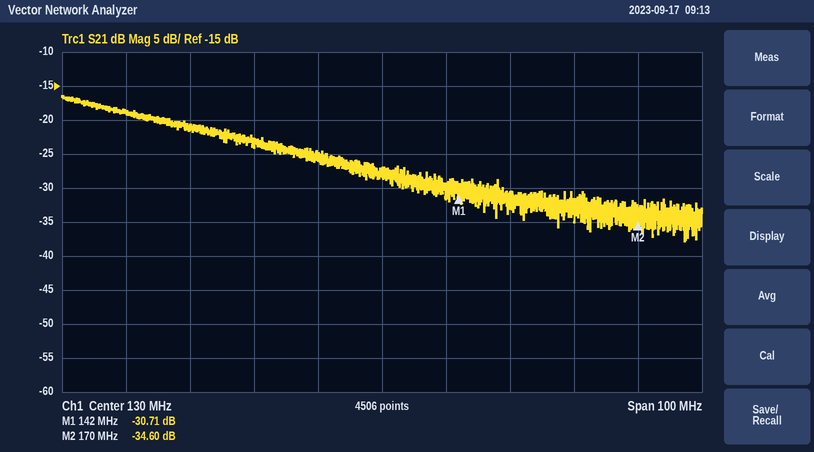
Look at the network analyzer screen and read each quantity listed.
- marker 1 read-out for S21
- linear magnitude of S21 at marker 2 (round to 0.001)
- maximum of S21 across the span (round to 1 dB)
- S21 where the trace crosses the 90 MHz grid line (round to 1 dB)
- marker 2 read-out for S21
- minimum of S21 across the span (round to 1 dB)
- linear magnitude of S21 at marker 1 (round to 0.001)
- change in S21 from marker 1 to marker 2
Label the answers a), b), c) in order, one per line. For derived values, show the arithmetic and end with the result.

a) -30.71 dB
b) 10^(-34.6/20) ≈ 0.019
c) -16 dB
d) -19 dB
e) -34.60 dB
f) -38 dB
g) 10^(-30.71/20) ≈ 0.029
h) -34.6 − (-30.71) = -3.89 dB
